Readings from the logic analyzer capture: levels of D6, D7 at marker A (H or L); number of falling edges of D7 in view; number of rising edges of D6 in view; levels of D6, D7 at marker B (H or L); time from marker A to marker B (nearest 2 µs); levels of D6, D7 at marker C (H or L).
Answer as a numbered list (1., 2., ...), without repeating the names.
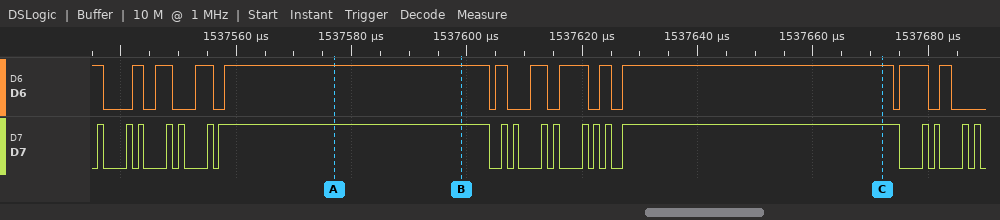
1. D6=H, D7=H
2. 19
3. 11
4. D6=H, D7=H
5. 22 µs
6. D6=H, D7=H
